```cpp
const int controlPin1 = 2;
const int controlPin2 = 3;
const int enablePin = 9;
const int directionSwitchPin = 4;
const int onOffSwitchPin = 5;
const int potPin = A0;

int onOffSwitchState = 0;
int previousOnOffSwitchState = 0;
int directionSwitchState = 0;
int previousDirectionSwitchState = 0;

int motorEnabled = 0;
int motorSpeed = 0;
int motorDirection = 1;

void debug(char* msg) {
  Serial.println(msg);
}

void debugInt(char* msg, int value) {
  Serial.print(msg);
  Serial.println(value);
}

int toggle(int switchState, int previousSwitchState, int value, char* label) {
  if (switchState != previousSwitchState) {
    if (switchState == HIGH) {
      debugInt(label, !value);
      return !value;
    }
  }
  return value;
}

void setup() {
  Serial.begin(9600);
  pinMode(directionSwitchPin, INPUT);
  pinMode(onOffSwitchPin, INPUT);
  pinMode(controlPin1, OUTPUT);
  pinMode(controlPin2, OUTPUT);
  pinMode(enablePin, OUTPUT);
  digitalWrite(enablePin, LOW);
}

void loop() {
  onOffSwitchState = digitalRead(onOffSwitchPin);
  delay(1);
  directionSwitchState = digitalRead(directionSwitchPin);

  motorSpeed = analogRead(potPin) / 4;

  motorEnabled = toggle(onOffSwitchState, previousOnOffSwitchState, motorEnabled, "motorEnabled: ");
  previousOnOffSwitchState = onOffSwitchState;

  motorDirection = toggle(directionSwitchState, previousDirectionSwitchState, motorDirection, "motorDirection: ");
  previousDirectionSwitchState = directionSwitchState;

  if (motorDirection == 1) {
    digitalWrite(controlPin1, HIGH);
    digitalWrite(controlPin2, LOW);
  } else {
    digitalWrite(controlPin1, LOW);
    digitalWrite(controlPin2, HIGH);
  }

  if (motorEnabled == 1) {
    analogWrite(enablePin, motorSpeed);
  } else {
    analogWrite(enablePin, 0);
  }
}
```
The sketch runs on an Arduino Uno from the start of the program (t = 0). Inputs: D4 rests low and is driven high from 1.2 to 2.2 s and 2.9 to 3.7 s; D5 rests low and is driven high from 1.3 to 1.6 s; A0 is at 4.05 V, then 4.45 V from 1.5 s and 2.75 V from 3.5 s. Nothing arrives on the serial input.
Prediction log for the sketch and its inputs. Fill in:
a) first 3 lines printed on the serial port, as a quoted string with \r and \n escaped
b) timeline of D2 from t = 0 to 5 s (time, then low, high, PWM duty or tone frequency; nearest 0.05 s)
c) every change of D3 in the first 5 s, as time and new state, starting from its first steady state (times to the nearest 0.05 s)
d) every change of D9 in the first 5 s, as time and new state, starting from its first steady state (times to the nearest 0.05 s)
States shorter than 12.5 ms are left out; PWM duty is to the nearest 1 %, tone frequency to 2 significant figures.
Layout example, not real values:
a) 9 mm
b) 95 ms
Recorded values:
a) "motorDirection: 0\r\nmotorEnabled: 1\r\nmotorDirection: 1\r\n"
b) 0 s high; 1.2 s low; 2.9 s high
c) 0 s low; 1.2 s high; 2.9 s low
d) 0 s low; 1.3 s PWM 81 %; 1.5 s PWM 89 %; 3.5 s PWM 55 %
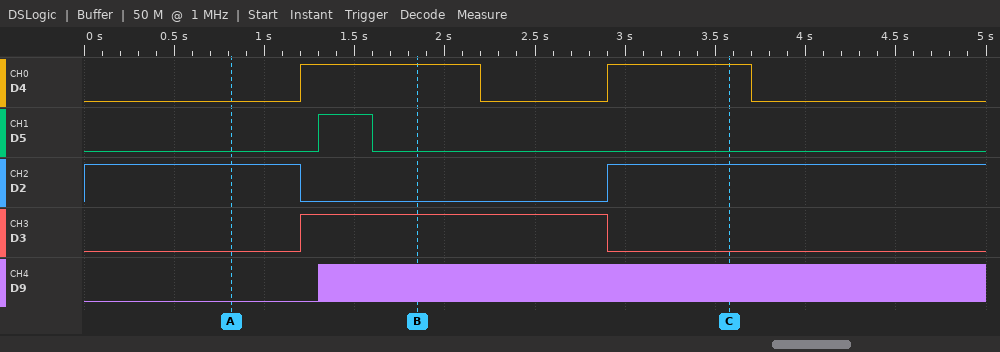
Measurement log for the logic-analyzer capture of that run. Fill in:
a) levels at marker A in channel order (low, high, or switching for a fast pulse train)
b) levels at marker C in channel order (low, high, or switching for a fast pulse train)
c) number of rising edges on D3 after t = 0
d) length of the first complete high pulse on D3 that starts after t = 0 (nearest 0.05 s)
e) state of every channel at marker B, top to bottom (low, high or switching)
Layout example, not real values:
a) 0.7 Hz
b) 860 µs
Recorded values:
a) D4 low, D5 low, D2 high, D3 low, D9 low
b) D4 high, D5 low, D2 high, D3 low, D9 switching
c) 1
d) 1.70 s
e) D4 high, D5 low, D2 low, D3 high, D9 switching
